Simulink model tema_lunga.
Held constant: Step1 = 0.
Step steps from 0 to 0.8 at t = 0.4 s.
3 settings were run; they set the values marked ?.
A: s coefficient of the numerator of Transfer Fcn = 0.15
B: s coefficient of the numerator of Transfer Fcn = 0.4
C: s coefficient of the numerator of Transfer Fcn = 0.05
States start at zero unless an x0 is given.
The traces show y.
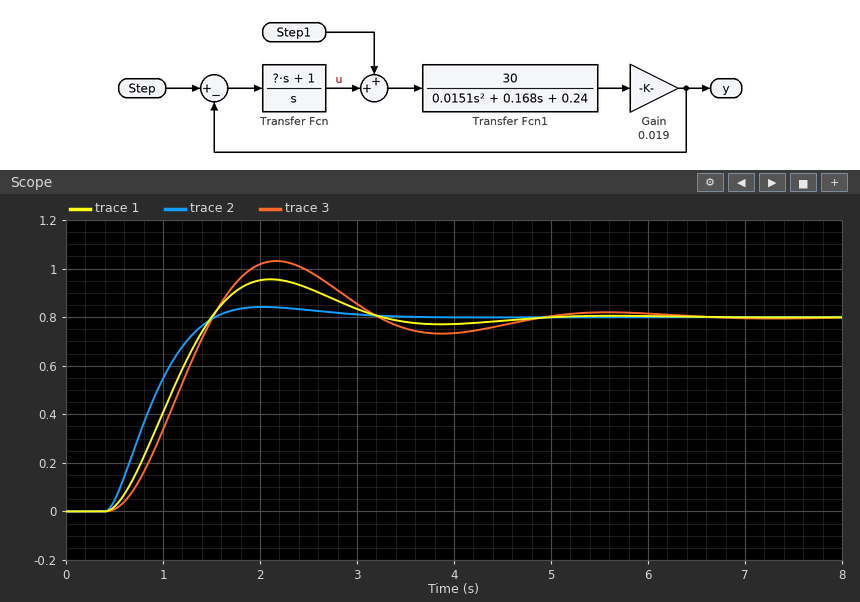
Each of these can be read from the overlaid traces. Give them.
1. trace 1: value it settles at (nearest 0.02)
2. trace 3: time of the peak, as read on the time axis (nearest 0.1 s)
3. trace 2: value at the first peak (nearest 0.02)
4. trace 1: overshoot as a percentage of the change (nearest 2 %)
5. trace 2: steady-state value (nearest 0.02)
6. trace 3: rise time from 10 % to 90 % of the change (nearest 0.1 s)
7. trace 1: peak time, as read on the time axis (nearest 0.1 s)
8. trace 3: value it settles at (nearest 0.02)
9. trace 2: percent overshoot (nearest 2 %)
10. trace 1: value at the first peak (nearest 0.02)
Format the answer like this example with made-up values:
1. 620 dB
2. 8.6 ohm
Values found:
1. 0.80
2. 2.2 s
3. 0.84
4. 20 %
5. 0.80
6. 0.7 s
7. 2.1 s
8. 0.80
9. 6 %
10. 0.96
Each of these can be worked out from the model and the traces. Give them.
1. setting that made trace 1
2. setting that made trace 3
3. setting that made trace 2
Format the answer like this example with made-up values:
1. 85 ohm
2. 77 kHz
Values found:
1. A
2. C
3. B
